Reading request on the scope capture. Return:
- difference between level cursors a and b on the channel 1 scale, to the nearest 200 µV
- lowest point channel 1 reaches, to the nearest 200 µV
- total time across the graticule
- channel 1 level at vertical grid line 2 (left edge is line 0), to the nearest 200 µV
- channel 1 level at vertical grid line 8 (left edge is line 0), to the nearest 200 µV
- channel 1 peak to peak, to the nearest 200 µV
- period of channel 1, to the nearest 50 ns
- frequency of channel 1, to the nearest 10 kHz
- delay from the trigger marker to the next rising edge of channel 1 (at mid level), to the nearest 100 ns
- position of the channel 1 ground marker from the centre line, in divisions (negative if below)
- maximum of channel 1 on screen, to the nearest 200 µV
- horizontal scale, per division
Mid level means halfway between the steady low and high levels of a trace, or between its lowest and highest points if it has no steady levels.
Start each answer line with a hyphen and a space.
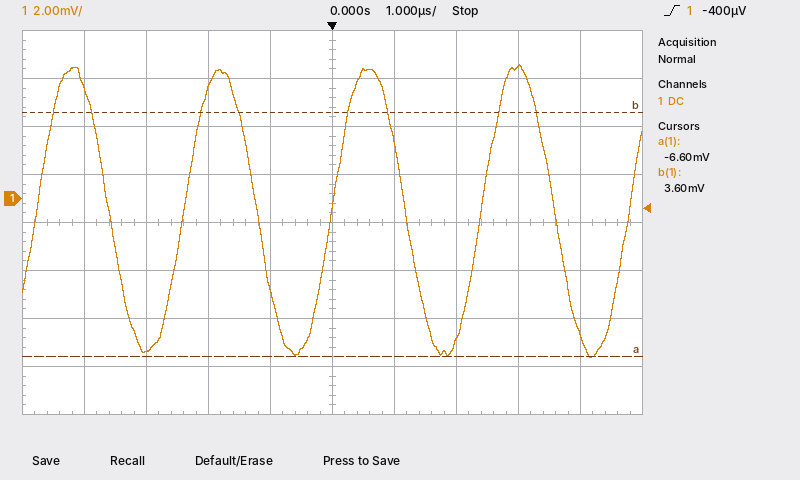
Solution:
- 10.2 mV
- -6.6 mV
- 10 µs
- -6.4 mV
- 5.4 mV
- 12.2 mV
- 2.40 µs
- 420 kHz
- 2.4 µs
- +0.5 div
- 5.6 mV
- 1 µs
